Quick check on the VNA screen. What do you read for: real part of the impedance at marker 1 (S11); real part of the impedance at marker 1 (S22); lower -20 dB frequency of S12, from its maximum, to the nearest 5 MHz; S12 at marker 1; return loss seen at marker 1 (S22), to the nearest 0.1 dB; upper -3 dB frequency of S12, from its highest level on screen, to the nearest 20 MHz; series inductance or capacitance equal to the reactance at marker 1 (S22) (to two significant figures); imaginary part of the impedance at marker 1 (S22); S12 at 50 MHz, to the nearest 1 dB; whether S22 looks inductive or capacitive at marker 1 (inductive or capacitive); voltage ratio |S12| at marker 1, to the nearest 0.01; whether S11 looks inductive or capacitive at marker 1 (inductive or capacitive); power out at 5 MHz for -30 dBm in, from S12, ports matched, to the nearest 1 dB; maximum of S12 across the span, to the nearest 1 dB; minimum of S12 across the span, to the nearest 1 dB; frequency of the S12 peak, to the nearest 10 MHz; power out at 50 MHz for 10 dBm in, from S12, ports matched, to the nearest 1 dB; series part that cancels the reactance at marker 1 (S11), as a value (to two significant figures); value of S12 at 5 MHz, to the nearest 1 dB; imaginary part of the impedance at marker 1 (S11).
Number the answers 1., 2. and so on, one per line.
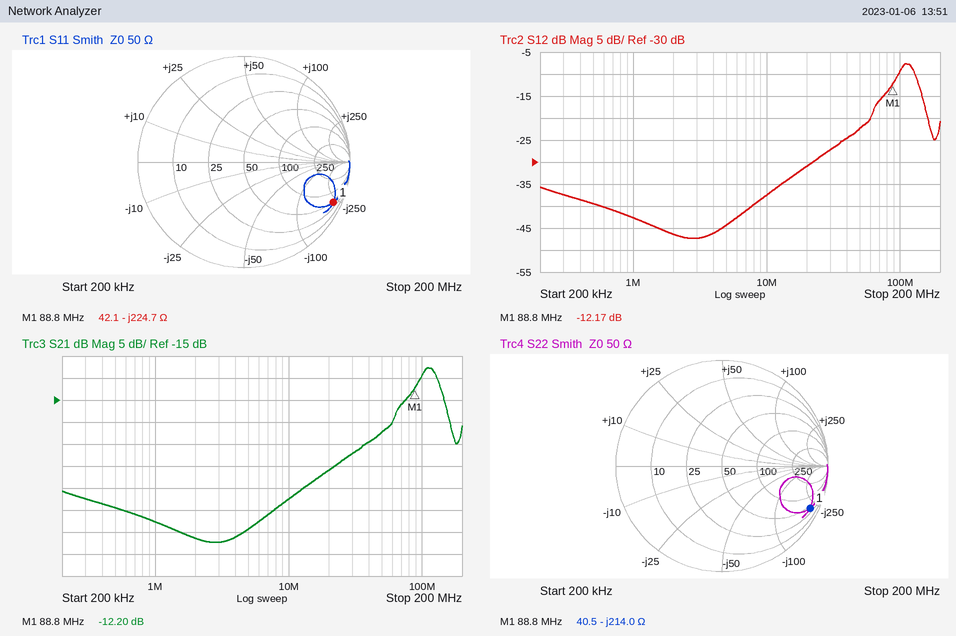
1. 42.1 Ω
2. 40.5 Ω
3. 30 MHz
4. -12.17 dB
5. 0.7 dB
6. 140 MHz
7. 8.4 pF
8. -214.0 Ω
9. -22 dB
10. capacitive
11. 0.25
12. capacitive
13. -74 dBm
14. -8 dB
15. -47 dB
16. 110 MHz
17. -12 dBm
18. 400 nH
19. -44 dB
20. -224.7 Ω
